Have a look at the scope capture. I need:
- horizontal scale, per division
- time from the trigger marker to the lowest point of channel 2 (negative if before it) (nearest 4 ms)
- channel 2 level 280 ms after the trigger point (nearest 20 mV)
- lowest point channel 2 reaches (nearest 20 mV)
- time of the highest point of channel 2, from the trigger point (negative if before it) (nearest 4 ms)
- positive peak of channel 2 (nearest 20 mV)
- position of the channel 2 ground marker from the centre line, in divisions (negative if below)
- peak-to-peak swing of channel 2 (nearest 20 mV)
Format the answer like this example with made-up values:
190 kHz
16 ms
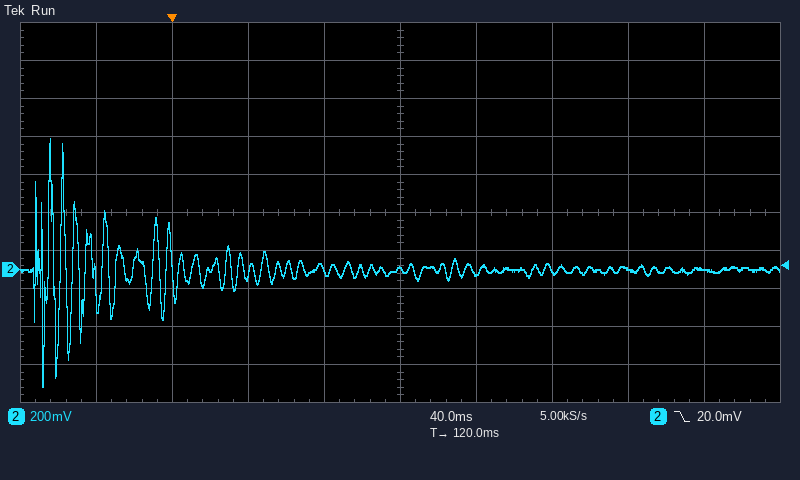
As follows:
40 ms
-68 ms
0 mV
-620 mV
-64 ms
680 mV
-1.5 div
1.30 V
